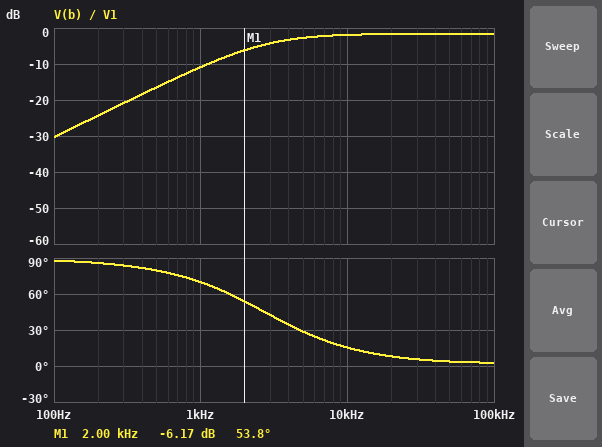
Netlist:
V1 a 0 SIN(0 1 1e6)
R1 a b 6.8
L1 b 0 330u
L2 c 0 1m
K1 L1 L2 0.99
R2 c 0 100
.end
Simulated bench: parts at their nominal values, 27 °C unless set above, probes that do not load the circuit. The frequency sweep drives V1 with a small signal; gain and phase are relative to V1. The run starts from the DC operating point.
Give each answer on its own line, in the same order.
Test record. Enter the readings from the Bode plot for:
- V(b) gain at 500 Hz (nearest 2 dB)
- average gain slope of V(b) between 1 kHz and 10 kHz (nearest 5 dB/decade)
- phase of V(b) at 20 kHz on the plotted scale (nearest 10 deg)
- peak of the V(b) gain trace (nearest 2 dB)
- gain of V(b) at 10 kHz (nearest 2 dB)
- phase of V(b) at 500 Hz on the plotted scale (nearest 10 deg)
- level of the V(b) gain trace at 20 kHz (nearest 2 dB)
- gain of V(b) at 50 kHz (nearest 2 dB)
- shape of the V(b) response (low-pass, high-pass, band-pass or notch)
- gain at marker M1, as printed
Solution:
-16 dB
10 dB/decade
10 deg
-2 dB
-2 dB
80 deg
-2 dB
-2 dB
high-pass
-6.17 dB
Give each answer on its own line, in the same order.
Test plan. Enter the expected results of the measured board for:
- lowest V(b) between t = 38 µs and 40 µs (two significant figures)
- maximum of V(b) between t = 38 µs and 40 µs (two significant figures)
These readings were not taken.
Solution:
-920 mV
920 mV
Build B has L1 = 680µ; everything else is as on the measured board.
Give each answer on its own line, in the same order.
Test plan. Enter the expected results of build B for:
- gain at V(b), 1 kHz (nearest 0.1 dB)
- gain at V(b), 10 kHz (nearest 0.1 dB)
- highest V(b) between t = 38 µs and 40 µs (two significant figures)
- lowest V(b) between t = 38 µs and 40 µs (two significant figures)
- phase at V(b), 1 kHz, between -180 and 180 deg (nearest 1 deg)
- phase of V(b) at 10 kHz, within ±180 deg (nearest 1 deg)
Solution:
-5.7 dB
-0.9 dB
960 mV
-960 mV
55 deg
8 deg
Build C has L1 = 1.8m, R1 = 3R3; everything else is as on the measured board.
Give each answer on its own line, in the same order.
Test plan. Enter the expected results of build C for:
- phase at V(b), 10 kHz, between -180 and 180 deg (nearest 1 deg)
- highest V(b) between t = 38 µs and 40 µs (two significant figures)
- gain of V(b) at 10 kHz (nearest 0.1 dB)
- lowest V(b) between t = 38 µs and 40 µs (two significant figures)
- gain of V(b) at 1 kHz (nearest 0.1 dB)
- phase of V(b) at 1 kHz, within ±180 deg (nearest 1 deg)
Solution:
2 deg
990 mV
-0.2 dB
-990 mV
-0.5 dB
16 deg
